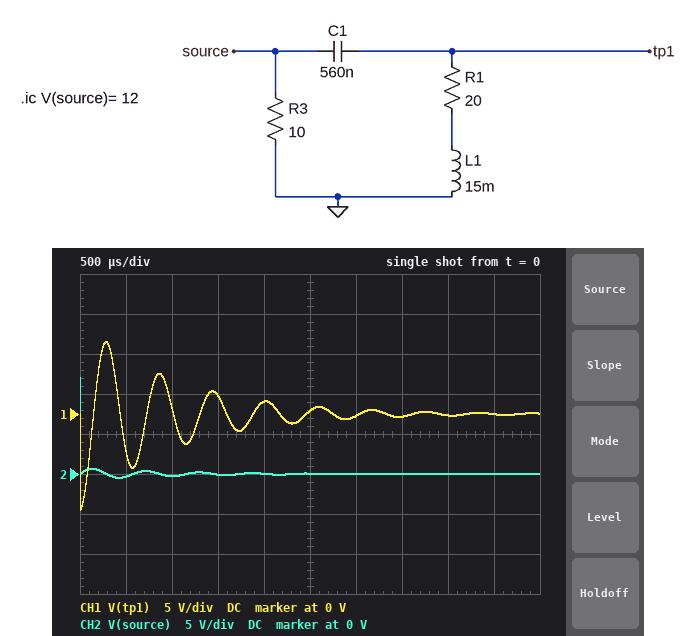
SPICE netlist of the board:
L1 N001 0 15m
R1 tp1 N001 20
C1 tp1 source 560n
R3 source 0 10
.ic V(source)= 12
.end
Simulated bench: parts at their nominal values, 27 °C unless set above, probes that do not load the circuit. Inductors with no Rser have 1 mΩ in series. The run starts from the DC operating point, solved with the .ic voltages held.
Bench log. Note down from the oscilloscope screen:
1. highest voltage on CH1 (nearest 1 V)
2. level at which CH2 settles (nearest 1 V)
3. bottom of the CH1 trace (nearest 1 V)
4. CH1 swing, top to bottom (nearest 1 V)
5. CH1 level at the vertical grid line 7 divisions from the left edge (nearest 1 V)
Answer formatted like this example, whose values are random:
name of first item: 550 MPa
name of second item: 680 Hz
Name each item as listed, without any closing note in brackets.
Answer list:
highest voltage on CH1: 9 V
level at which CH2 settles: 0 V
bottom of the CH1 trace: -12 V
CH1 swing, top to bottom: 21 V
CH1 level at the vertical grid line 7 divisions from the left edge: 0 V
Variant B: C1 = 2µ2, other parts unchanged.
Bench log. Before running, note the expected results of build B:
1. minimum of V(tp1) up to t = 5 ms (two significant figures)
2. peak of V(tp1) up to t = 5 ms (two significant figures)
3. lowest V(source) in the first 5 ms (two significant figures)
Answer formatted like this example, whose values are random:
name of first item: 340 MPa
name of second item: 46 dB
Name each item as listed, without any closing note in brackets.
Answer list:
minimum of V(tp1) up to t = 5 ms: -12 V
peak of V(tp1) up to t = 5 ms: 6.8 V
lowest V(source) in the first 5 ms: -630 mV
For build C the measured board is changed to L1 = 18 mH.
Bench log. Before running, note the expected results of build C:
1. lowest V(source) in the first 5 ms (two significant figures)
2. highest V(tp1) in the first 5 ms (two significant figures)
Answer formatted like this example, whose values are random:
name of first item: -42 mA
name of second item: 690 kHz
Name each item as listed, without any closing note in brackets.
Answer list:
lowest V(source) in the first 5 ms: -450 mV
highest V(tp1) in the first 5 ms: 9.2 V
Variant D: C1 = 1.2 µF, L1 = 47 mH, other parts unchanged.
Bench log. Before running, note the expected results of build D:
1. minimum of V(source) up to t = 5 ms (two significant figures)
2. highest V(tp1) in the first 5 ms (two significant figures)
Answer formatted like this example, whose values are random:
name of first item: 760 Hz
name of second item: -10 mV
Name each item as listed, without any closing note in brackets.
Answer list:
minimum of V(source) up to t = 5 ms: -430 mV
highest V(tp1) in the first 5 ms: 9.5 V
